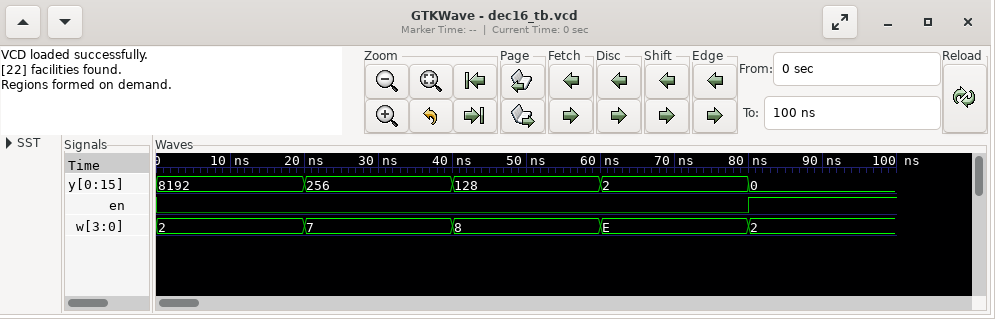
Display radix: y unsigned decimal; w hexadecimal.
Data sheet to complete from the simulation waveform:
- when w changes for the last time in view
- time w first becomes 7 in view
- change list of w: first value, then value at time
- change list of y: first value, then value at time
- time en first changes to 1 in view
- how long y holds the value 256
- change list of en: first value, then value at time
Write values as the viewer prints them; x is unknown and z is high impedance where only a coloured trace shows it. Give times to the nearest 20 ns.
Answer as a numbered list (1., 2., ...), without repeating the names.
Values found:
1. 80 ns
2. 20 ns
3. 2, 7 at 20 ns, 8 at 40 ns, E at 60 ns, 2 at 80 ns
4. 8192, 256 at 20 ns, 128 at 40 ns, 2 at 60 ns, 0 at 80 ns
5. 80 ns
6. 20 ns
7. 0, 1 at 80 ns
